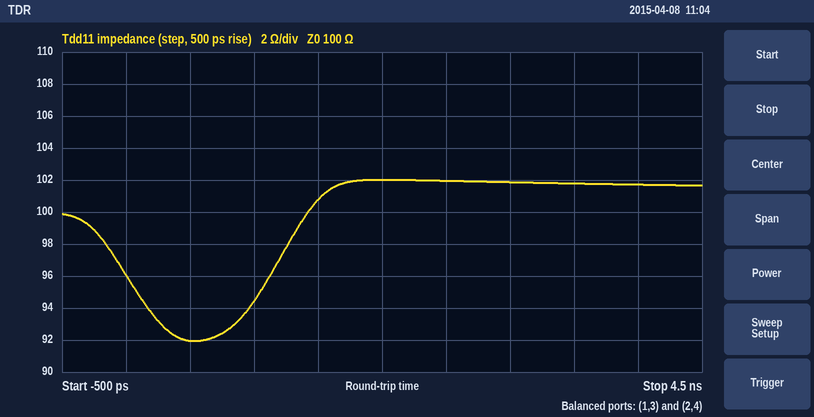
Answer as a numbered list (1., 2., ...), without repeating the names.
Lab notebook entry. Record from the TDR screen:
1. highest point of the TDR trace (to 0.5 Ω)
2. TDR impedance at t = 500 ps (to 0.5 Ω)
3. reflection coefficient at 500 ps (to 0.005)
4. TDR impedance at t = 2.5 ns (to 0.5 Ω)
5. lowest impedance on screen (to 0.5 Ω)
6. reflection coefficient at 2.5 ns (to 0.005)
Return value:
1. 102.0 Ω
2. 92.0 Ω
3. -0.040
4. 102.0 Ω
5. 92.0 Ω
6. +0.010
